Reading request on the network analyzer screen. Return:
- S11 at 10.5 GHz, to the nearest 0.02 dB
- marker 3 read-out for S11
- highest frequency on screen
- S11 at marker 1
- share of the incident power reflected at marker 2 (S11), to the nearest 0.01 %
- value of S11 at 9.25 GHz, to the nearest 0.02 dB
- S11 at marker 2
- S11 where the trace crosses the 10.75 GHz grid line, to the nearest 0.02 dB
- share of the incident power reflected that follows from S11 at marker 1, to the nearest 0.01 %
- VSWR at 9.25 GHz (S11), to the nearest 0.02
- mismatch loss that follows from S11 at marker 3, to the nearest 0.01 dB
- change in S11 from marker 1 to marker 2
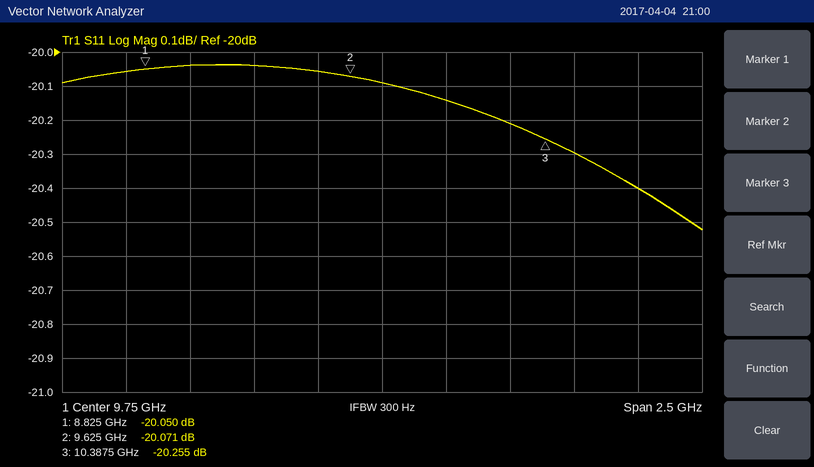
-20.30 dB
-20.255 dB
11 GHz
-20.050 dB
0.98 %
-20.04 dB
-20.071 dB
-20.40 dB
0.99 %
1.22
0.04 dB
-0.021 dB
